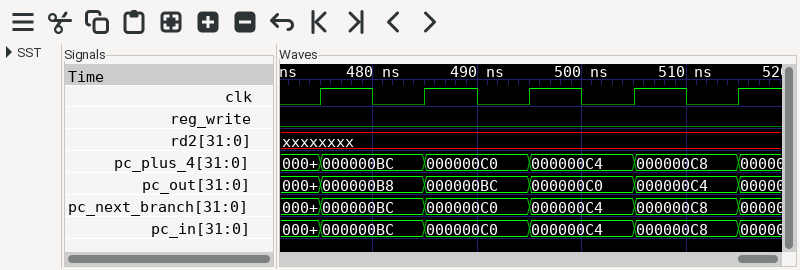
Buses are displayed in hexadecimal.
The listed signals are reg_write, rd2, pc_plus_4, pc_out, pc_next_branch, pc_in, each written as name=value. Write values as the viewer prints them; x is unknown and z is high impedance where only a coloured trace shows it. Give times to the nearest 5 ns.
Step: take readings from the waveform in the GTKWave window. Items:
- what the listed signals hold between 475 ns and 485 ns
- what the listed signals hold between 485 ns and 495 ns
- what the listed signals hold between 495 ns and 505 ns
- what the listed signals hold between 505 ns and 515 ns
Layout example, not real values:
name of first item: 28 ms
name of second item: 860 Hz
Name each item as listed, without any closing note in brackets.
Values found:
what the listed signals hold between 475 ns and 485 ns: reg_write=0, rd2=xxxxxxxx, pc_plus_4=000000BC, pc_out=000000B8, pc_next_branch=000000BC, pc_in=000000BC
what the listed signals hold between 485 ns and 495 ns: reg_write=0, rd2=xxxxxxxx, pc_plus_4=000000C0, pc_out=000000BC, pc_next_branch=000000C0, pc_in=000000C0
what the listed signals hold between 495 ns and 505 ns: reg_write=0, rd2=xxxxxxxx, pc_plus_4=000000C4, pc_out=000000C0, pc_next_branch=000000C4, pc_in=000000C4
what the listed signals hold between 505 ns and 515 ns: reg_write=0, rd2=xxxxxxxx, pc_plus_4=000000C8, pc_out=000000C4, pc_next_branch=000000C8, pc_in=000000C8
